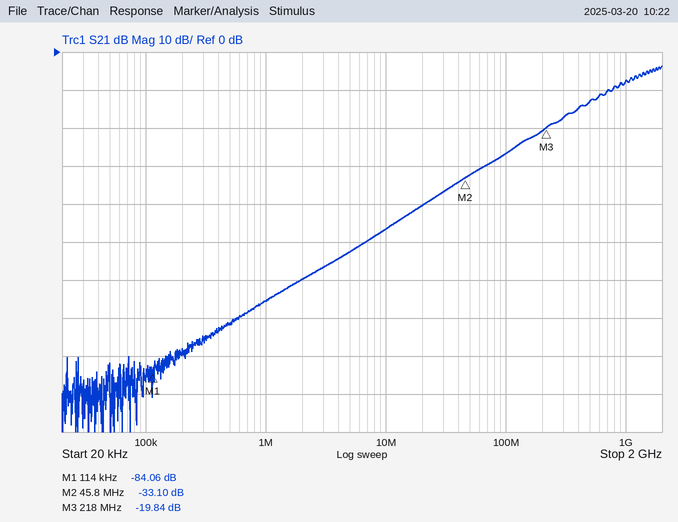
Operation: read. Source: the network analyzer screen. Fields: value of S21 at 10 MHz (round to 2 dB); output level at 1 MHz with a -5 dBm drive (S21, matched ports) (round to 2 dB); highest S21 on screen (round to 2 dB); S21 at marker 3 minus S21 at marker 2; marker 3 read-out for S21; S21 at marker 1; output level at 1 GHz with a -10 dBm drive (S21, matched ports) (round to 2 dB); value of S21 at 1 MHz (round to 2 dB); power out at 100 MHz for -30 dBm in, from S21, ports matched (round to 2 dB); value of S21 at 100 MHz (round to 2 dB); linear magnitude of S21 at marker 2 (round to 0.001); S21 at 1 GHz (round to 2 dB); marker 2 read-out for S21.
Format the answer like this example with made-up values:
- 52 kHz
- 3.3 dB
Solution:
- -46 dB
- -70 dBm
- -4 dB
- 13.26 dB
- -19.84 dB
- -84.06 dB
- -18 dBm
- -66 dB
- -56 dBm
- -26 dB
- 0.022
- -8 dB
- -33.10 dB
